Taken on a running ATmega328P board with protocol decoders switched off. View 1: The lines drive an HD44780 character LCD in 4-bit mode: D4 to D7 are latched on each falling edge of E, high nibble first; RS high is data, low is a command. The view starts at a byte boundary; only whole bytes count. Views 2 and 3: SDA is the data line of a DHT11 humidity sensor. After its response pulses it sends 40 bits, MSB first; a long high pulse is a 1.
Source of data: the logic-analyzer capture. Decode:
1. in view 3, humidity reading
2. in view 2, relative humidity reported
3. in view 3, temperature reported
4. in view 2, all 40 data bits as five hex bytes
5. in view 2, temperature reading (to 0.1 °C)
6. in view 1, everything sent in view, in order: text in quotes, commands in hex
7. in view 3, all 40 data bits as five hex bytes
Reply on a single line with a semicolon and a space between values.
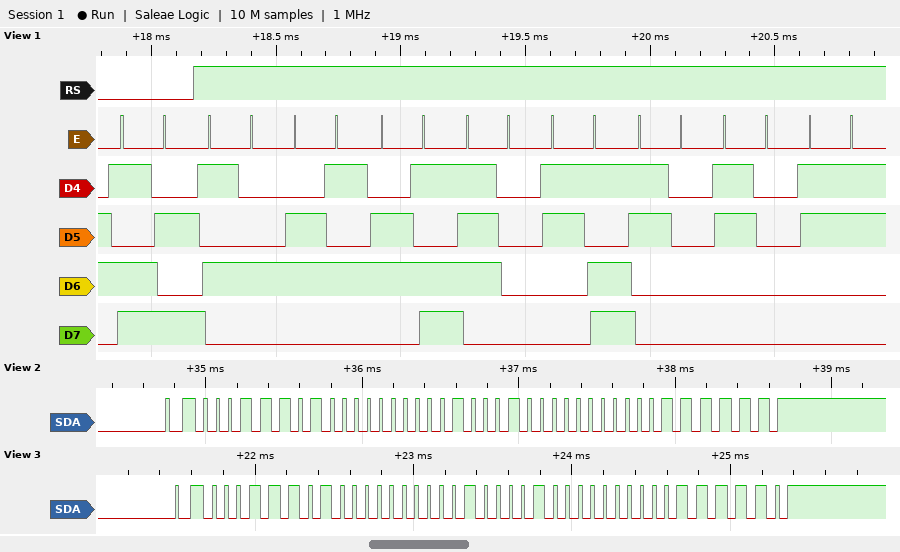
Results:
29 %; 29 %; 33.0 °C; 1D 00 22 00 3F; 34.0 °C; 0xDA "Temp=003"; 1D 00 21 00 3E
